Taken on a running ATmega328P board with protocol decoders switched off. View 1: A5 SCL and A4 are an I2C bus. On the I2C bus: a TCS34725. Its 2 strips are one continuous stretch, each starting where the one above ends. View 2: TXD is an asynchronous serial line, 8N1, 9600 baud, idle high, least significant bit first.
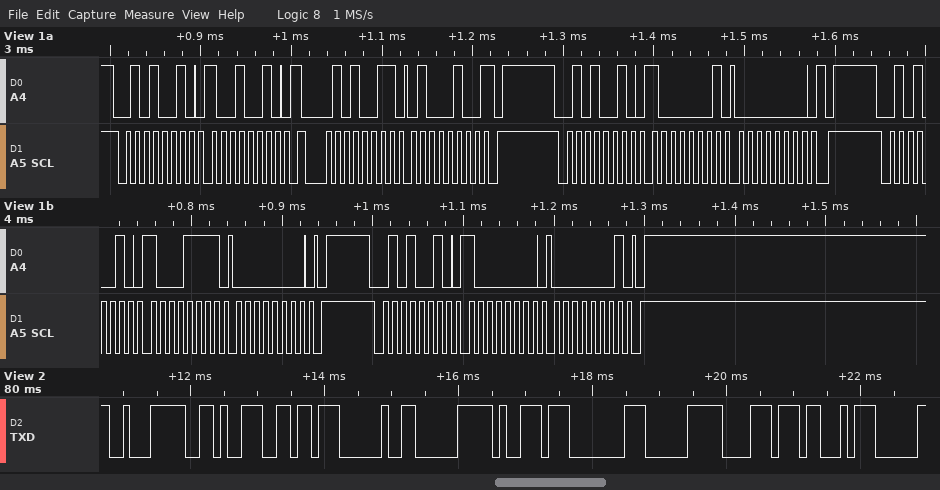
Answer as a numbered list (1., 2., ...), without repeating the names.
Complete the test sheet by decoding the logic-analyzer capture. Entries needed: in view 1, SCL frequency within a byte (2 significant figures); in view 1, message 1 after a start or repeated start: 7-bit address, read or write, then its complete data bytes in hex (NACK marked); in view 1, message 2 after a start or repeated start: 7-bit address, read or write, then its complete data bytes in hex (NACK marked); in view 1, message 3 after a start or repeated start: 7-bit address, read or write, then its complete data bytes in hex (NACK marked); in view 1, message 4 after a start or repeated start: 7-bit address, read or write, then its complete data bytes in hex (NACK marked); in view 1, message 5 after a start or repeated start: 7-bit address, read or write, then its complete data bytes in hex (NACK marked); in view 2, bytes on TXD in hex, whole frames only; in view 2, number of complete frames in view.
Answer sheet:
1. 100 kHz
2. 0x29 write: 92
3. 0x29 read: 44 NACK
4. 0x29 write: 81 00
5. 0x29 write: 8F 00
6. 0x29 write: 80 01
7. E2 96 B6 20 E0 B9 80 E0 B8 A3
8. 10
